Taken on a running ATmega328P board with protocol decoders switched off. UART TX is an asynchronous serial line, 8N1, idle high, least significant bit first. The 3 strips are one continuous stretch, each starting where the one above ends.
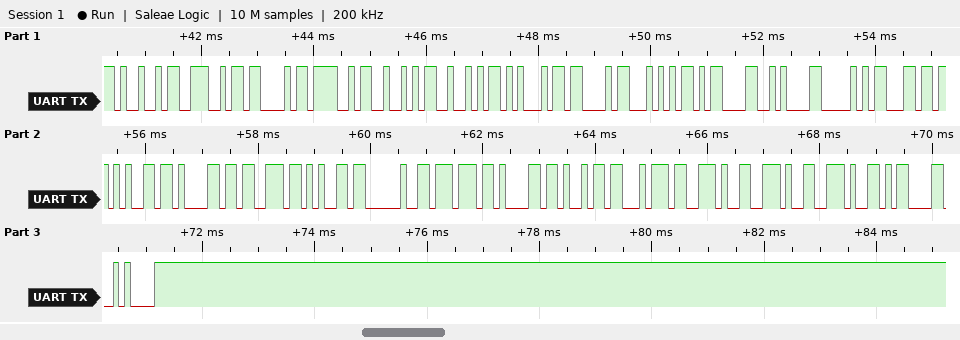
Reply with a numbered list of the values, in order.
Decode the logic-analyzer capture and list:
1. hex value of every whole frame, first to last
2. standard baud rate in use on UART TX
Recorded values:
1. 49 4E 43 4F 52 52 45 43 54 0D 0A 50 6C 65 61 73 65 20 77 61 69 74 2E 2E 2E 0D 0A
2. 9600 baud
